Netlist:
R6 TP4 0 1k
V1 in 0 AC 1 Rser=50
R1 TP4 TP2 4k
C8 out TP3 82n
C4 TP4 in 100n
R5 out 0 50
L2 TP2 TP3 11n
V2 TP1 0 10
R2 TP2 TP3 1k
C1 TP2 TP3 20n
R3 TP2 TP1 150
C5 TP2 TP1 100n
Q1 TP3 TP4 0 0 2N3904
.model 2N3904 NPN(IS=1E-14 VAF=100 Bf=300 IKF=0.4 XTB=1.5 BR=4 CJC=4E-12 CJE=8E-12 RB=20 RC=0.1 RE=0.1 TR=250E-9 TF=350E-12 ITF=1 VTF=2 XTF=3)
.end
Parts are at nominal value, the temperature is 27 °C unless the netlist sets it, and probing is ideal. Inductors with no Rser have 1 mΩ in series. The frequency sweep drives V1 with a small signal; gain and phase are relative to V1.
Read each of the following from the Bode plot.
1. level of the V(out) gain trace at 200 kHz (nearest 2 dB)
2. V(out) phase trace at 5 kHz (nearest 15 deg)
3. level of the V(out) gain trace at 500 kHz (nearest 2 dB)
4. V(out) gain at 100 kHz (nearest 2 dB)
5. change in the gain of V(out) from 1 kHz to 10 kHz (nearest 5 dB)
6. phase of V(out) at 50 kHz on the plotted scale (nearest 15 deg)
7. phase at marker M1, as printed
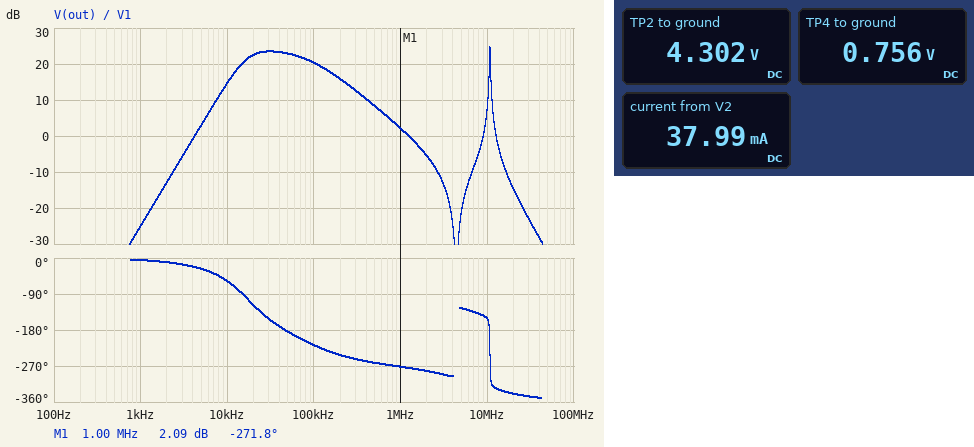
16 dB
-30 deg
8 dB
20 dB
40 dB
-180 deg
-271.8 deg
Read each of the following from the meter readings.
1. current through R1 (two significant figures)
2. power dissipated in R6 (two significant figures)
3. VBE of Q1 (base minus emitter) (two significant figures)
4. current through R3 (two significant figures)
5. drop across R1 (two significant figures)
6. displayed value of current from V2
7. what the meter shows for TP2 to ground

890 µA
570 µW
760 mV
38 mA
3.5 V
37.99 mA
4.302 V
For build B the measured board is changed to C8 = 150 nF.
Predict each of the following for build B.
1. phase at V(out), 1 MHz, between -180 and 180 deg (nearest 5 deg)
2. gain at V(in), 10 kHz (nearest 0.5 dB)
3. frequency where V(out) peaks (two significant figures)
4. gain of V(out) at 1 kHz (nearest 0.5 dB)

85 deg
-1.5 dB
28 kHz
-19.5 dB
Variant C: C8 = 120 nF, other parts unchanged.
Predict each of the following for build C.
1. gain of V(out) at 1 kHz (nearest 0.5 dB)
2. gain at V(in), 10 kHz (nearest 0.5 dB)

-21.5 dB
-1.5 dB
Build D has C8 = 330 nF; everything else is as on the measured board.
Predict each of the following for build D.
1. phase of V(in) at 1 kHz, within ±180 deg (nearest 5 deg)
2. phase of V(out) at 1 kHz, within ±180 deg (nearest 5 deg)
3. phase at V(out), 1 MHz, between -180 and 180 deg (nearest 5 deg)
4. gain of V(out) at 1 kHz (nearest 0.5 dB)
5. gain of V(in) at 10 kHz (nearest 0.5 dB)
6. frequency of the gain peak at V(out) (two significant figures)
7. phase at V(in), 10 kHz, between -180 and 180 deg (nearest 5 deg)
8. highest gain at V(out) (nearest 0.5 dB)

0 deg
-10 deg
85 deg
-13.0 dB
-1.5 dB
27 kHz
-15 deg
25.5 dB
